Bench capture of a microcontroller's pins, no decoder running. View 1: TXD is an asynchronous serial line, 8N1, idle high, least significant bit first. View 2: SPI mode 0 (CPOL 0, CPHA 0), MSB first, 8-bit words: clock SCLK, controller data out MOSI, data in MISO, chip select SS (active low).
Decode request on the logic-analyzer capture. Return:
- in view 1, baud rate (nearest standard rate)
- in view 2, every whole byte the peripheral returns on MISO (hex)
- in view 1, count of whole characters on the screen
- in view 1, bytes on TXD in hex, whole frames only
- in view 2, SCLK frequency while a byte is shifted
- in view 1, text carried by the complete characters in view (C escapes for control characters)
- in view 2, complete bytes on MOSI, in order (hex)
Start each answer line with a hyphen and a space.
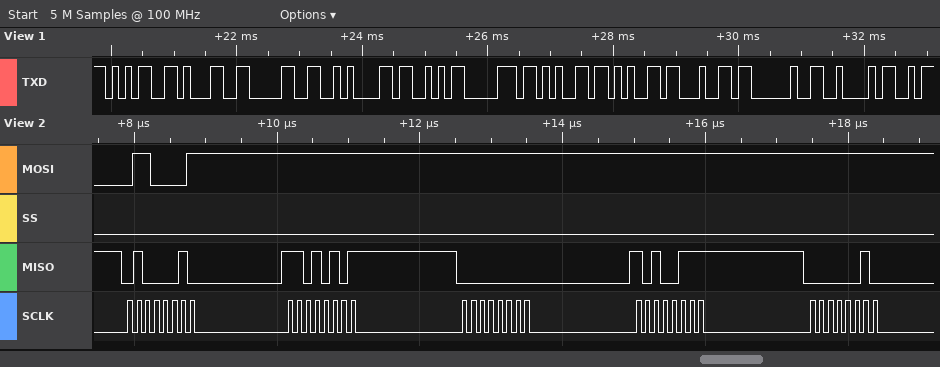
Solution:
- 9600 baud
- 42 D5 00 A7 02
- 11
- 35 31 30 0A 53 70 65 65 64 20 42
- 8 MHz
- "510\nSpeed B"
- 61 FF FF FF FF
